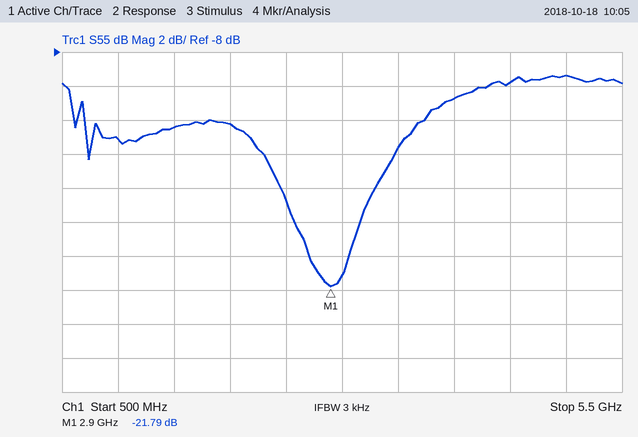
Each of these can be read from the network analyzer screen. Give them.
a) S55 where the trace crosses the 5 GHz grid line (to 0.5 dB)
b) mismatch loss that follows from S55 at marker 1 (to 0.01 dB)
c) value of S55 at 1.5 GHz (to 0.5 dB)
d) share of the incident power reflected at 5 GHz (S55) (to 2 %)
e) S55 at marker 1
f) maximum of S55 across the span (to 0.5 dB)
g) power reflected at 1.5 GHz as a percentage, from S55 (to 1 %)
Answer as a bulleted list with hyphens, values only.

- -9.5 dB
- 0.03 dB
- -12.5 dB
- 12 %
- -21.79 dB
- -9.5 dB
- 6 %
